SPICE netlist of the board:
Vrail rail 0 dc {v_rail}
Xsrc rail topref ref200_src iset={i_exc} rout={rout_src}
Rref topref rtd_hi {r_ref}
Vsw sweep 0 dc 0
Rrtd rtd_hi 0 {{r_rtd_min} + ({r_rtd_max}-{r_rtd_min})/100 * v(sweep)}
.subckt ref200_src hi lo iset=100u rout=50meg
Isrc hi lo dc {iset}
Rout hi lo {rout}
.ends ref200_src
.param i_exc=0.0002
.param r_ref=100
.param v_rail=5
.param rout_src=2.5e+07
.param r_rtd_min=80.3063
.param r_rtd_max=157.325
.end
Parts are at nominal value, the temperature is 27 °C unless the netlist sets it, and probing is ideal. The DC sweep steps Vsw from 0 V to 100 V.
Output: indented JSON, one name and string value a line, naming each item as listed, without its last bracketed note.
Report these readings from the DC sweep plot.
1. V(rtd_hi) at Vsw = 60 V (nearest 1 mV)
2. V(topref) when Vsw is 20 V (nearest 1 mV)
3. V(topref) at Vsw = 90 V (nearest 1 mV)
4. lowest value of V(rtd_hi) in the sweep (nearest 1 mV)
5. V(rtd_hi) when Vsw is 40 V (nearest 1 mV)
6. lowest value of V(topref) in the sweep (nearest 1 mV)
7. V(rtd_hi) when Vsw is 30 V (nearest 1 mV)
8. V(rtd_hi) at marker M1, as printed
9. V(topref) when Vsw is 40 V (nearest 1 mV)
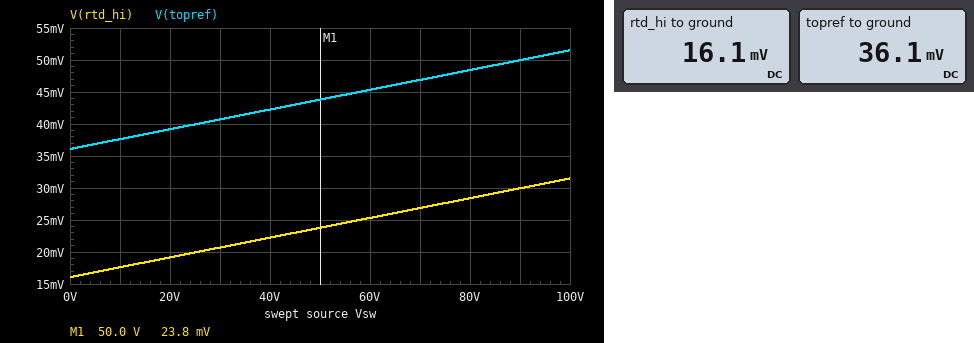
{
  "V(rtd_hi) at Vsw = 60 V": "25 mV",
  "V(topref) when Vsw is 20 V": "39 mV",
  "V(topref) at Vsw = 90 V": "50 mV",
  "lowest value of V(rtd_hi) in the sweep": "16 mV",
  "V(rtd_hi) when Vsw is 40 V": "22 mV",
  "lowest value of V(topref) in the sweep": "36 mV",
  "V(rtd_hi) when Vsw is 30 V": "21 mV",
  "V(rtd_hi) at marker M1, as printed": "23.8 mV",
  "V(topref) when Vsw is 40 V": "42 mV"
}
